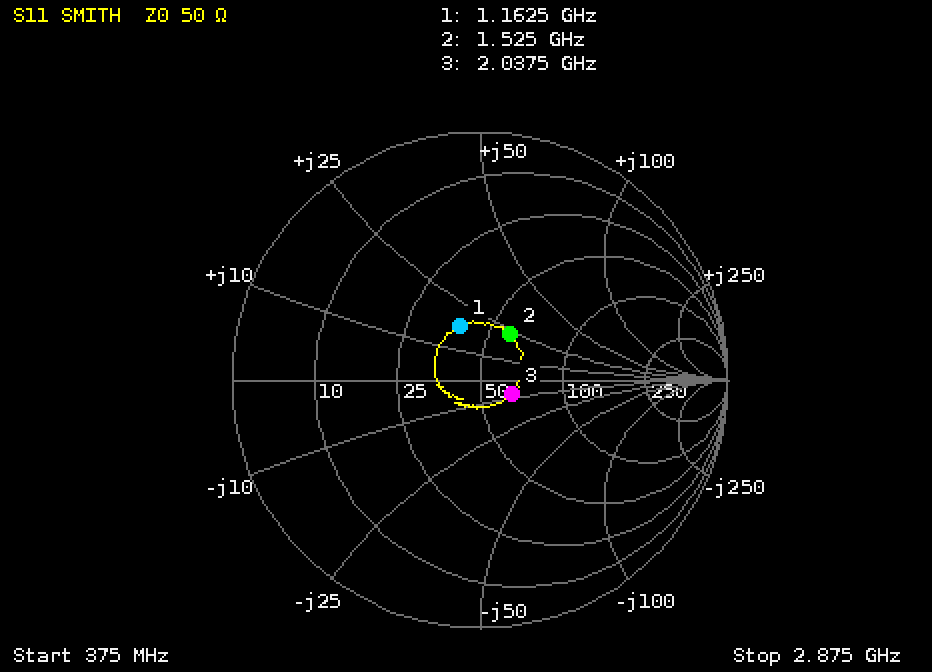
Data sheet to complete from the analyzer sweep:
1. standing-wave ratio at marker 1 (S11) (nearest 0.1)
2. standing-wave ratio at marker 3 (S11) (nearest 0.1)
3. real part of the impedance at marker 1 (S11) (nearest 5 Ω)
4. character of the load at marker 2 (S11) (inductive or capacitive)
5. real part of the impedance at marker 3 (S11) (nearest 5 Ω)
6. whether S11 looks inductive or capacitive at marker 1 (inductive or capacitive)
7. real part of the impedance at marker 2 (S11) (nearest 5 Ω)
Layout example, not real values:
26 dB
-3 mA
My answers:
1.6
1.3
40 Ω
inductive
65 Ω
inductive
60 Ω
